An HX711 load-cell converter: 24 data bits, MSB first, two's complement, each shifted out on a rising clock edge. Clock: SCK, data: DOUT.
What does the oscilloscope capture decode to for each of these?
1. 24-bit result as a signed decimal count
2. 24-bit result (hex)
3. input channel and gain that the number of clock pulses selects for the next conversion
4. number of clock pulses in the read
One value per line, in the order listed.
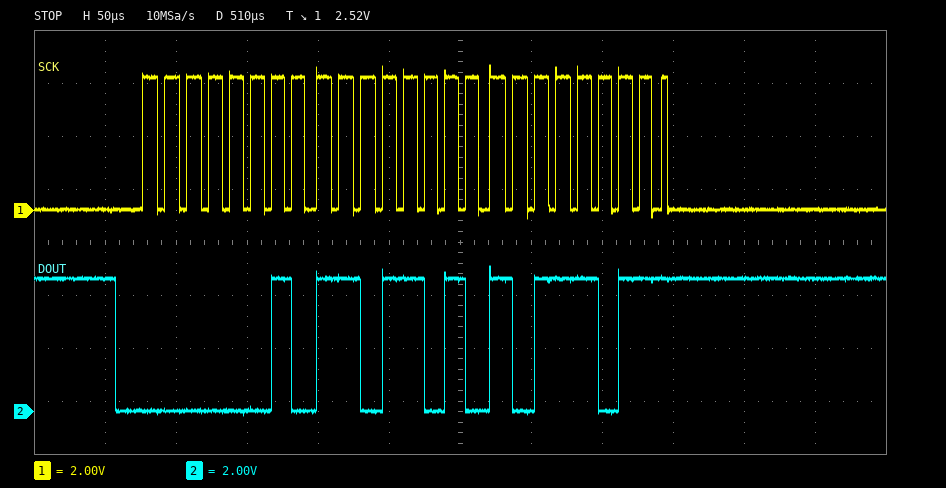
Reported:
187067
0x02DABB
channel A, gain 128
25
